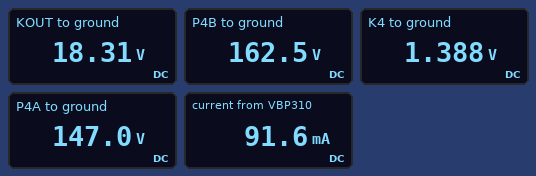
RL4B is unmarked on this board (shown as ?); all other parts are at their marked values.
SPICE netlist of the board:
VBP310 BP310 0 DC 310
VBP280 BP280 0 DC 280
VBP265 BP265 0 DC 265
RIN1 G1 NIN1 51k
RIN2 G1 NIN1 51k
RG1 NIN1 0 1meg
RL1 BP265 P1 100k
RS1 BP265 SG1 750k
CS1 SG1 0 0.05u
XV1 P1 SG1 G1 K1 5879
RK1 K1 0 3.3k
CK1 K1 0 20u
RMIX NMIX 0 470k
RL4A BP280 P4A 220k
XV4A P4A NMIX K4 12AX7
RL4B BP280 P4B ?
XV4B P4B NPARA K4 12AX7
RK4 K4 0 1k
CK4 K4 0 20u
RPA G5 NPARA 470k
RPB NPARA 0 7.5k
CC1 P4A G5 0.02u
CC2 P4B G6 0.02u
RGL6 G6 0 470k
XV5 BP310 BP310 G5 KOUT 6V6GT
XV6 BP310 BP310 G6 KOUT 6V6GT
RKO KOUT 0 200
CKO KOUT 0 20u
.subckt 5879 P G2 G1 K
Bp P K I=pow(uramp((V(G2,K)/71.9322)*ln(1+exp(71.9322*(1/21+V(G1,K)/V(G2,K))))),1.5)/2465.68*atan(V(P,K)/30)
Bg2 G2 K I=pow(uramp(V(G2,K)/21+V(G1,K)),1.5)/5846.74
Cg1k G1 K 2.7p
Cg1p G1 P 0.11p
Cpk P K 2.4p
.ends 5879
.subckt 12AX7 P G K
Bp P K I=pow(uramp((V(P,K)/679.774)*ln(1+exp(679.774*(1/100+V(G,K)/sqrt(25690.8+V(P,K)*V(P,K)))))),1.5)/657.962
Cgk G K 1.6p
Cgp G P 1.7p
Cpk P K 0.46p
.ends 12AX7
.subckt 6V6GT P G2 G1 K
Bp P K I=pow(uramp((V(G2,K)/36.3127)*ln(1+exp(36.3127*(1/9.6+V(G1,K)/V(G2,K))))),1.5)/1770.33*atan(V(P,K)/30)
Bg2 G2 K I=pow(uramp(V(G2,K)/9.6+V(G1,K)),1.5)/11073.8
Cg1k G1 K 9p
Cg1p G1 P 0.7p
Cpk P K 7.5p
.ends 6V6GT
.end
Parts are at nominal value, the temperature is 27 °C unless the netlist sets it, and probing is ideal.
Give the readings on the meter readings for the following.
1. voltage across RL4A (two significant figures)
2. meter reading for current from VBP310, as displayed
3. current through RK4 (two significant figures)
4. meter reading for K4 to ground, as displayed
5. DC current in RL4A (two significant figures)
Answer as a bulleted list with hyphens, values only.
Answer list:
- 130 V
- 91.6 mA
- 1.4 mA
- 1.388 V
- 600 µA
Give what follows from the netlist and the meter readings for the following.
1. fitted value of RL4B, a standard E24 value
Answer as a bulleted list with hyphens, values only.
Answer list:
- 150 kΩ
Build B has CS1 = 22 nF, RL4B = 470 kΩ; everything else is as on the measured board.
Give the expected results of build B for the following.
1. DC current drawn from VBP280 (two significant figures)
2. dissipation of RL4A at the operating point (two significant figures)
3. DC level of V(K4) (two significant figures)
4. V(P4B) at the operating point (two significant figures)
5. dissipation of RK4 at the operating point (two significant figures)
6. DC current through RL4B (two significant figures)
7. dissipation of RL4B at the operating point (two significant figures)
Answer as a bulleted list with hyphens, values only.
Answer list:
- 1.1 mA
- 110 mW
- 1.1 V
- 96 V
- 1.2 mW
- 390 µA
- 72 mW
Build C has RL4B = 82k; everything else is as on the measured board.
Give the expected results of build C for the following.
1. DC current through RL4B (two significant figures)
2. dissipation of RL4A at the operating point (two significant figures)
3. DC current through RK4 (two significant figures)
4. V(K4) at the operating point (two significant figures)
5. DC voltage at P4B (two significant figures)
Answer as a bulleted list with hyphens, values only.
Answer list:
- 1.0 mA
- 66 mW
- 1.6 mA
- 1.6 V
- 200 V
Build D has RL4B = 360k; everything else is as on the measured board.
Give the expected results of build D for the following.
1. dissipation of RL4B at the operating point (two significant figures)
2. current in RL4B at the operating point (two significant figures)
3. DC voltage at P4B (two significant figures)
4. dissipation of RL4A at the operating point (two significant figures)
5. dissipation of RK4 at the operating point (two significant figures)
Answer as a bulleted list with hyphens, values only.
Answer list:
- 80 mW
- 470 µA
- 110 V
- 100 mW
- 1.3 mW
